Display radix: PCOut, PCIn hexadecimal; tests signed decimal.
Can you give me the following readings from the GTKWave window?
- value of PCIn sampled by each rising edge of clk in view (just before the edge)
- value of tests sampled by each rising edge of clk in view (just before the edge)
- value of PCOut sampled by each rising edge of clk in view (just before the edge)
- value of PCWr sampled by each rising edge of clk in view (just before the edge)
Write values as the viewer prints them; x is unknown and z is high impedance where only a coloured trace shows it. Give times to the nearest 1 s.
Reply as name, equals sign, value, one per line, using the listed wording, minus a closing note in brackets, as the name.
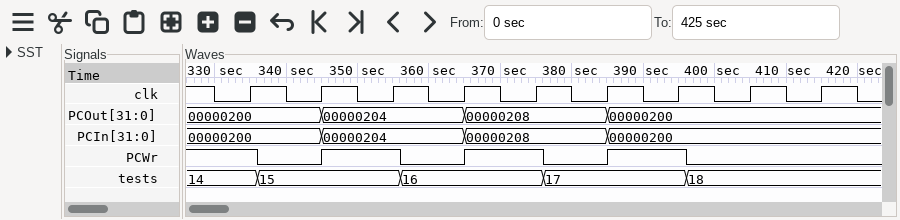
value of PCIn sampled by each rising edge of clk in view = 00000200, 00000200, 00000204, 00000204, 00000208, 00000208, 00000200, 00000200, 00000200
value of tests sampled by each rising edge of clk in view = 14, 15, 15, 16, 16, 17, 17, 18, 18
value of PCOut sampled by each rising edge of clk in view = 00000200, 00000200, 00000204, 00000204, 00000208, 00000208, 00000200, 00000200, 00000200
value of PCWr sampled by each rising edge of clk in view = 1 0 1 0 1 0 1 0 0
